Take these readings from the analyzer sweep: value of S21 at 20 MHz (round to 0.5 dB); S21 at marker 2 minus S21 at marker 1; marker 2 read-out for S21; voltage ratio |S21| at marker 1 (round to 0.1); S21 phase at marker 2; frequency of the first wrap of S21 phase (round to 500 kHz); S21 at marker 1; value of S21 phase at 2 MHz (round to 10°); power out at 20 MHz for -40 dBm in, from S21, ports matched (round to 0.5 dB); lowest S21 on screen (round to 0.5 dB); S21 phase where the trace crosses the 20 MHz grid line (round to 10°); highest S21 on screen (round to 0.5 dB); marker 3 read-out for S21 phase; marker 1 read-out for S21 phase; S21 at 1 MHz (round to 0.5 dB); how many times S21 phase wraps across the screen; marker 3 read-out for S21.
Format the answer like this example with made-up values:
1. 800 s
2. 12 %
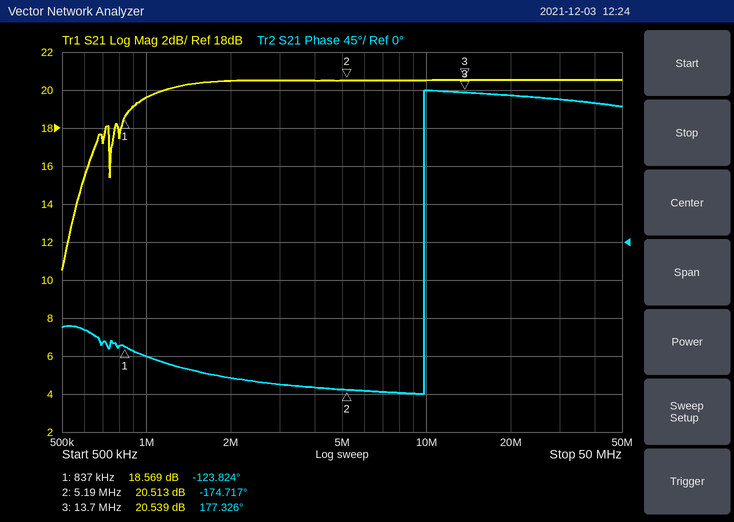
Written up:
1. 20.5 dB
2. 1.944 dB
3. 20.513 dB
4. 8.5
5. -174.717°
6. 10.0 MHz
7. 18.569 dB
8. -160°
9. -19.5 dBm
10. 10.5 dB
11. 170°
12. 20.5 dB
13. 177.326°
14. -123.824°
15. 19.5 dB
16. 1
17. 20.539 dB
